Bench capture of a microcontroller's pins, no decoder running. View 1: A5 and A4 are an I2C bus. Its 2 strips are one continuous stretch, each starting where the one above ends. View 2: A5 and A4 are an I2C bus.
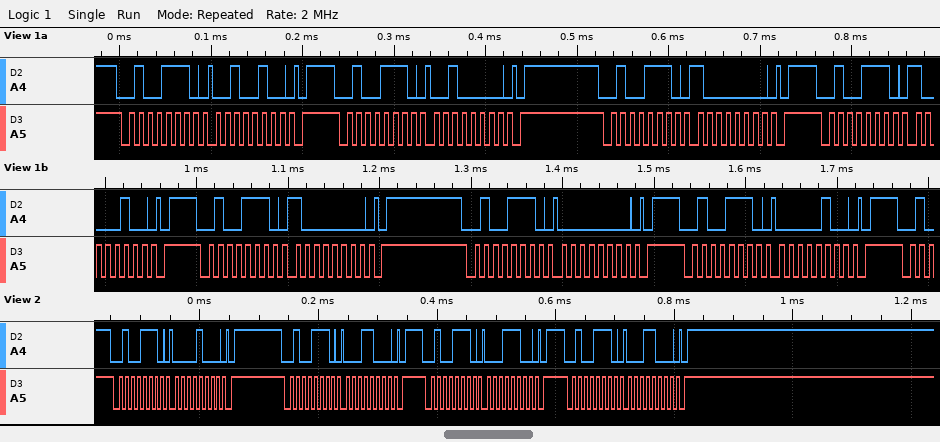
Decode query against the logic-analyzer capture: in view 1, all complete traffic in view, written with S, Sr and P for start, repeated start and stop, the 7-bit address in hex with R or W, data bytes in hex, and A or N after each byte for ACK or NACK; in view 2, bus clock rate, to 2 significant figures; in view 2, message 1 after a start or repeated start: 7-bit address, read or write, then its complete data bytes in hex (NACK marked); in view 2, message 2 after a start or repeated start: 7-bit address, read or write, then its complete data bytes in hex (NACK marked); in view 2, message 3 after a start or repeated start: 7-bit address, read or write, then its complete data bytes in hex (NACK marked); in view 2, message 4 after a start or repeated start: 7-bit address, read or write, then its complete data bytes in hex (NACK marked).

S 27W A 24 A P S 27W A 20 A P S 27W A 80 A P S 27W A 84 A P S 27W A 80 A P S 27W A 00 A P S 27W A 04 A P
100 kHz
0x27 write: 08
0x27 write: 18
0x27 write: 1C
0x27 write: 18
